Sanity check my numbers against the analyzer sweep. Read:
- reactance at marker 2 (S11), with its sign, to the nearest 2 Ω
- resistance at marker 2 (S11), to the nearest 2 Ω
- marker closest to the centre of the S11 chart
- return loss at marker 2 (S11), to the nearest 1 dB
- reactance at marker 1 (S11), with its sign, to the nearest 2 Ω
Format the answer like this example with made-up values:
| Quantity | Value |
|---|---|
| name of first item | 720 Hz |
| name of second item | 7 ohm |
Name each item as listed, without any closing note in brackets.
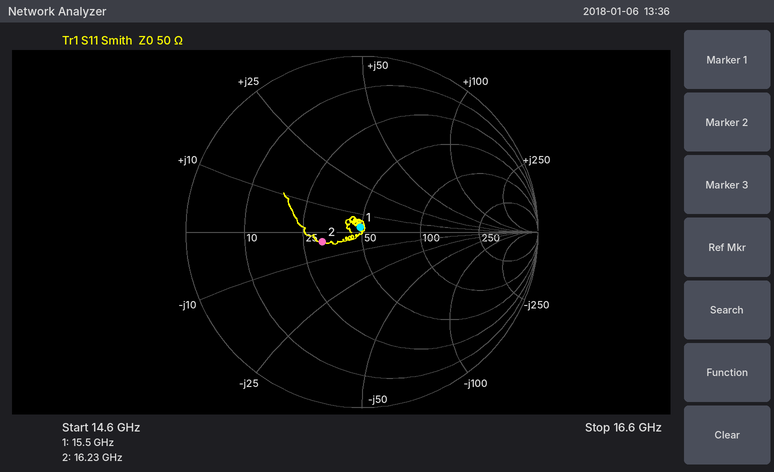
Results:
| Quantity | Value |
|---|---|
| reactance at marker 2 (S11), with its sign, to the nearest 2 Ω | -4 Ω |
| resistance at marker 2 (S11), to the nearest 2 Ω | 32 Ω |
| marker closest to the centre of the S11 chart | marker 1 |
| return loss at marker 2 (S11), to the nearest 1 dB | 13 dB |
| reactance at marker 1 (S11), with its sign, to the nearest 2 Ω | +2 Ω |
